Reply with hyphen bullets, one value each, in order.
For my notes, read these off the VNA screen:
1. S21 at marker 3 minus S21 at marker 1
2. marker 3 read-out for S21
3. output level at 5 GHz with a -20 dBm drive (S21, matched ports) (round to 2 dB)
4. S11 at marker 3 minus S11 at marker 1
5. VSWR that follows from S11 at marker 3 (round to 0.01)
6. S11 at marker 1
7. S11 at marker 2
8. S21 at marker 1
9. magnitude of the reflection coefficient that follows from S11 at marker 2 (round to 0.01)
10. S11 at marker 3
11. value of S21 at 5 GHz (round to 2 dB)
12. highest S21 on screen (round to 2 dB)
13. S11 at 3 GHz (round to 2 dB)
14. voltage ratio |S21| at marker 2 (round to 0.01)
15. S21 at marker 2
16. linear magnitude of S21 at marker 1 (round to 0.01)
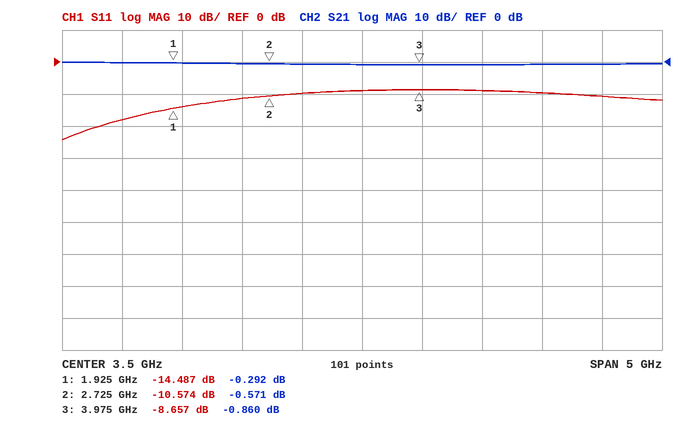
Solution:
- -0.568 dB
- -0.860 dB
- -20 dBm
- 5.830 dB
- 2.17
- -14.487 dB
- -10.574 dB
- -0.292 dB
- 0.30
- -8.657 dB
- 0 dB
- 0 dB
- -10 dB
- 0.94
- -0.571 dB
- 0.97
